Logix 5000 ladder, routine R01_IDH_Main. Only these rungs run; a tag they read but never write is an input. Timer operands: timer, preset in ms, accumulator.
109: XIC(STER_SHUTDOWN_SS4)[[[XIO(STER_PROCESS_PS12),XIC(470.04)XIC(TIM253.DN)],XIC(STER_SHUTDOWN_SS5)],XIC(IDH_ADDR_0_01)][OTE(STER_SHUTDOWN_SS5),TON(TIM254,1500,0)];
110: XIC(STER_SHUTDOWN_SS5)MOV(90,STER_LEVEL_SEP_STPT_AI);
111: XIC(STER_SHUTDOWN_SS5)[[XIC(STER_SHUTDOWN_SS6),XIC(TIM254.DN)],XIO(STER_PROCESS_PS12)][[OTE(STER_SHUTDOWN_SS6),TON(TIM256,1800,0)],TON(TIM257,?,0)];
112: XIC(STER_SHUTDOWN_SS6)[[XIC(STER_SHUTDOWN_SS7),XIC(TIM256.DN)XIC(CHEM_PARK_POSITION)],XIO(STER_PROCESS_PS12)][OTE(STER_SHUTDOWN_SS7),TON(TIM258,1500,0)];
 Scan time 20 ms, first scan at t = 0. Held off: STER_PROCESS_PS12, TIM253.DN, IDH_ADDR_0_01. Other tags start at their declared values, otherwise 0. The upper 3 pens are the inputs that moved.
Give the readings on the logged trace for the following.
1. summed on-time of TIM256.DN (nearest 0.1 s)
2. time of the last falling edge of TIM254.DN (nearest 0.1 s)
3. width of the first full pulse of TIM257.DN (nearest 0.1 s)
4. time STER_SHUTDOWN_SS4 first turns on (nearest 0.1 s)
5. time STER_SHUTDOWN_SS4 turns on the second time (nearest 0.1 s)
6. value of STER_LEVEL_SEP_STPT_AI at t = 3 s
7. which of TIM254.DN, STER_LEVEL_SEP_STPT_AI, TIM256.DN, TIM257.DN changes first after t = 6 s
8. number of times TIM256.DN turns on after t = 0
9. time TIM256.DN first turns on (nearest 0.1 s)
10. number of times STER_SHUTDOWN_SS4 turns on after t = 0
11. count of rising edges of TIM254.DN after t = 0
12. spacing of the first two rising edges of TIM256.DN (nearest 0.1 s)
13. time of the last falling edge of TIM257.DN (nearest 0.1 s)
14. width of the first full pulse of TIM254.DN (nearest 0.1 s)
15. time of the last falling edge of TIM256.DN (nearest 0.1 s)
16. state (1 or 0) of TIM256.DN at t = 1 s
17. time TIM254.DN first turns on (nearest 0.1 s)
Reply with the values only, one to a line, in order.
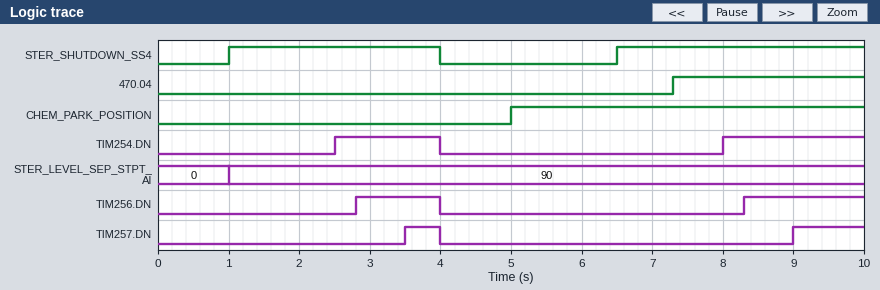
2.9 s
4.0 s
0.5 s
1.0 s
6.5 s
90
TIM254.DN
2
2.8 s
2
2
5.5 s
4.0 s
1.5 s
4.0 s
0
2.5 s
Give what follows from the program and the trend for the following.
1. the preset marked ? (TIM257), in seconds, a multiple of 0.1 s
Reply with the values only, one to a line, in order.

2.5 s
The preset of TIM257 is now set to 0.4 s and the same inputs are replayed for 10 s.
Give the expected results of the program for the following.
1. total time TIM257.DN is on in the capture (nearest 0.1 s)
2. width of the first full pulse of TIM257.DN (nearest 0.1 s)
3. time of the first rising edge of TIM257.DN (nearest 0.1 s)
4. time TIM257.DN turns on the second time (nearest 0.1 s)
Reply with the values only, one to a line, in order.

5.7 s
2.6 s
1.4 s
6.9 s
